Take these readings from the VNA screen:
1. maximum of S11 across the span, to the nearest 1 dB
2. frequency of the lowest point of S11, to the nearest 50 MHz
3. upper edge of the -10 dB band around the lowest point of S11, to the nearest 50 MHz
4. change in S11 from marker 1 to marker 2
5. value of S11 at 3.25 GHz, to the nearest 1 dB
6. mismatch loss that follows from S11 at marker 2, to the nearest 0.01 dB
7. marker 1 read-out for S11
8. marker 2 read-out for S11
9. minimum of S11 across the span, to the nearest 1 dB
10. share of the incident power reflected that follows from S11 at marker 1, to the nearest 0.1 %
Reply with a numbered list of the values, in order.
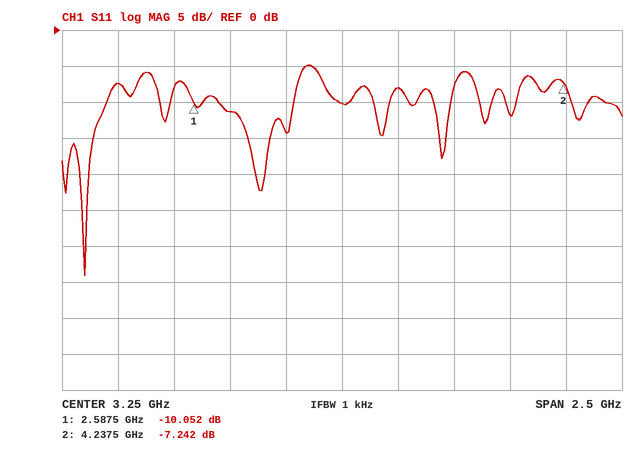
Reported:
1. -5 dB
2. 2.10 GHz
3. 2.20 GHz
4. 2.810 dB
5. -10 dB
6. 0.91 dB
7. -10.052 dB
8. -7.242 dB
9. -34 dB
10. 9.9 %
